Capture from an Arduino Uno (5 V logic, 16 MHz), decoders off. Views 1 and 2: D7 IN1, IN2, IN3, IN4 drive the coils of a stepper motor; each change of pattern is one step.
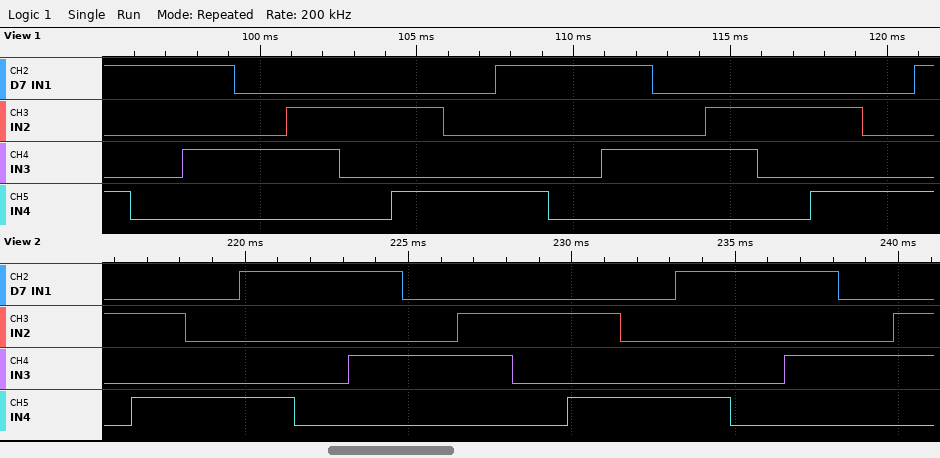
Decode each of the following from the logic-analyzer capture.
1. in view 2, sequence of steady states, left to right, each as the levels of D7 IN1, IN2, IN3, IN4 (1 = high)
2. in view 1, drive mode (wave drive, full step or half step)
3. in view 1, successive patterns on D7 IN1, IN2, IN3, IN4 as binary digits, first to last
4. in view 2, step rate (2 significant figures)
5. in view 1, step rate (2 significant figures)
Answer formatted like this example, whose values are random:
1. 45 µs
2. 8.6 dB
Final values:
1. 0100 0101 0001 1001 1000 1010 0010 0110 0100 0101 0001 1001 1000 1010 0010 0110
2. half step
3. 1001 1000 1010 0010 0110 0100 0101 0001 1001 1000 1010 0010 0110 0100 0101 0001 1001
4. 600 steps/s
5. 600 steps/s
